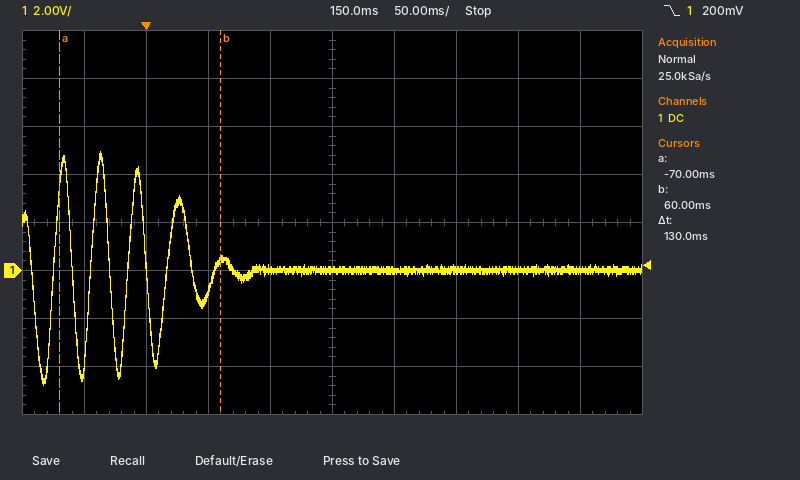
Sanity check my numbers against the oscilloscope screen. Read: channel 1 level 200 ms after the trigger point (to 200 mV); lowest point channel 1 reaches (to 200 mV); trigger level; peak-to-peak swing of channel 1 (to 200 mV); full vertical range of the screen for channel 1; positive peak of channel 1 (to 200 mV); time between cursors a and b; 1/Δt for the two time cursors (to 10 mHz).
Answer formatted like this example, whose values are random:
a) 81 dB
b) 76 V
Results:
a) 0.0 V
b) -4.8 V
c) 200 mV
d) 9.8 V
e) 16 V
f) 5.0 V
g) 130 ms
h) 7.69 Hz
